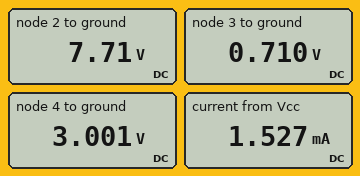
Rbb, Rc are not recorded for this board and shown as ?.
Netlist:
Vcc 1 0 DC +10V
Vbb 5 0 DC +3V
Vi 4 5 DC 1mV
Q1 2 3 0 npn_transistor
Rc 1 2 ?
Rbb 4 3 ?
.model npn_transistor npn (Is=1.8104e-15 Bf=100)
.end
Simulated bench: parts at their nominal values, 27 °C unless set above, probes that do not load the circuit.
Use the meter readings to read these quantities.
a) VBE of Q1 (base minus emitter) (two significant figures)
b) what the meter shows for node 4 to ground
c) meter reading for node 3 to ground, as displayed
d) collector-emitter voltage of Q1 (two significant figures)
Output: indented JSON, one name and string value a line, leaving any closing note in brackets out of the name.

{
  "VBE of Q1 (base minus emitter)": "710 mV",
  "what the meter shows for node 4 to ground": "3.001 V",
  "meter reading for node 3 to ground, as displayed": "0.710 V",
  "collector-emitter voltage of Q1": "7.7 V"
}
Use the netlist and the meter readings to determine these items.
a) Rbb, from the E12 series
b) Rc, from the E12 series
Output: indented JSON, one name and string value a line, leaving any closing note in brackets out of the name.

{
  "Rbb, from the E12 series": "150 kΩ",
  "Rc, from the E12 series": "1.5 kΩ"
}
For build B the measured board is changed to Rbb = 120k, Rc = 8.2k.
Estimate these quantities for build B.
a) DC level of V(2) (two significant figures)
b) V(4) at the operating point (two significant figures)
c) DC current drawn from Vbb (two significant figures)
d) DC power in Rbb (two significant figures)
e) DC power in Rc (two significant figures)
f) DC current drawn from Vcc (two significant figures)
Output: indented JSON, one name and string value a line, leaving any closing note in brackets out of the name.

{
  "DC level of V(2)": "130 mV",
  "V(4) at the operating point": "3.0 V",
  "DC current drawn from Vbb": "19 µA",
  "DC power in Rbb": "44 µW",
  "DC power in Rc": "12 mW",
  "DC current drawn from Vcc": "1.2 mA"
}
